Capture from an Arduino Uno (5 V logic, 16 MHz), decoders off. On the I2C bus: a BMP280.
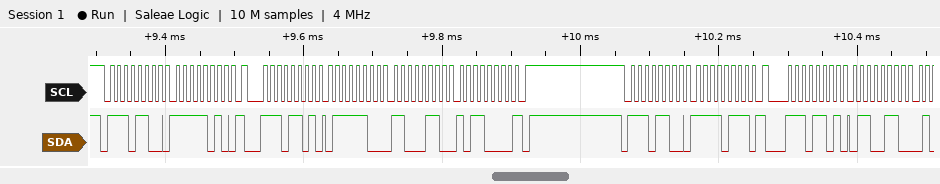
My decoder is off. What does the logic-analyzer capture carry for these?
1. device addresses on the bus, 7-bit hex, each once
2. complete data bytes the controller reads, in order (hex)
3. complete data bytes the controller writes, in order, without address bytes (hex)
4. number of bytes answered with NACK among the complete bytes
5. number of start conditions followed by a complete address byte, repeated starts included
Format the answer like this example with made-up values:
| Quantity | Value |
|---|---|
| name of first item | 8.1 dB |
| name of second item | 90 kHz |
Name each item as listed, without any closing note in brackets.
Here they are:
| Quantity | Value |
|---|---|
| device addresses on the bus, 7-bit hex, each once | 0x76 |
| complete data bytes the controller reads, in order | 7C C6 B0 66 |
| complete data bytes the controller writes, in order, without address bytes | FA F7 |
| number of bytes answered with NACK among the complete bytes | 1 |
| number of start conditions followed by a complete address byte, repeated starts included | 4 |
